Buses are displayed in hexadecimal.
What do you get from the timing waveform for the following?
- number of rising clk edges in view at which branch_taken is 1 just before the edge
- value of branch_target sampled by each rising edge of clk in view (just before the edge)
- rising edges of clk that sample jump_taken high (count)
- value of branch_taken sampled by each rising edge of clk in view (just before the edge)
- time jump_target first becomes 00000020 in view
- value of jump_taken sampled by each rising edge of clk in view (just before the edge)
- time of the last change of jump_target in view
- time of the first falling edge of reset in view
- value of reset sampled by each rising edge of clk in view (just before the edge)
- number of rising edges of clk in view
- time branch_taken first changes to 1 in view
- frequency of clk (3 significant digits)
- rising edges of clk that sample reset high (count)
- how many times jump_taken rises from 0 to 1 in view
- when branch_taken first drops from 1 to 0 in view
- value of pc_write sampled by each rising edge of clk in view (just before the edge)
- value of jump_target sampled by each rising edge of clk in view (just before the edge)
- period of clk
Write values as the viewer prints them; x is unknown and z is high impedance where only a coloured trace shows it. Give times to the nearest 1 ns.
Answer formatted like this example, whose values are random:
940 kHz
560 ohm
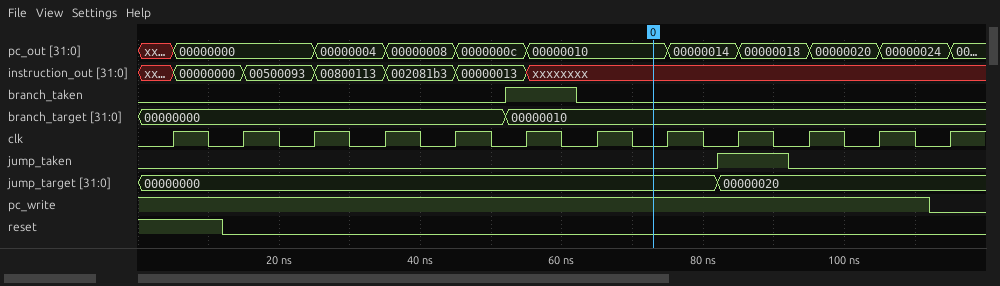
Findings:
1
00000000, 00000000, 00000000, 00000000, 00000000, 00000010, 00000010, 00000010, 00000010, 00000010, 00000010, 00000010
1
0 0 0 0 0 1 0 0 0 0 0 0
82 ns
0 0 0 0 0 0 0 0 1 0 0 0
82 ns
12 ns
1 0 0 0 0 0 0 0 0 0 0 0
12
52 ns
100 MHz
1
1
62 ns
1 1 1 1 1 1 1 1 1 1 1 0
00000000, 00000000, 00000000, 00000000, 00000000, 00000000, 00000000, 00000000, 00000020, 00000020, 00000020, 00000020
10 ns
